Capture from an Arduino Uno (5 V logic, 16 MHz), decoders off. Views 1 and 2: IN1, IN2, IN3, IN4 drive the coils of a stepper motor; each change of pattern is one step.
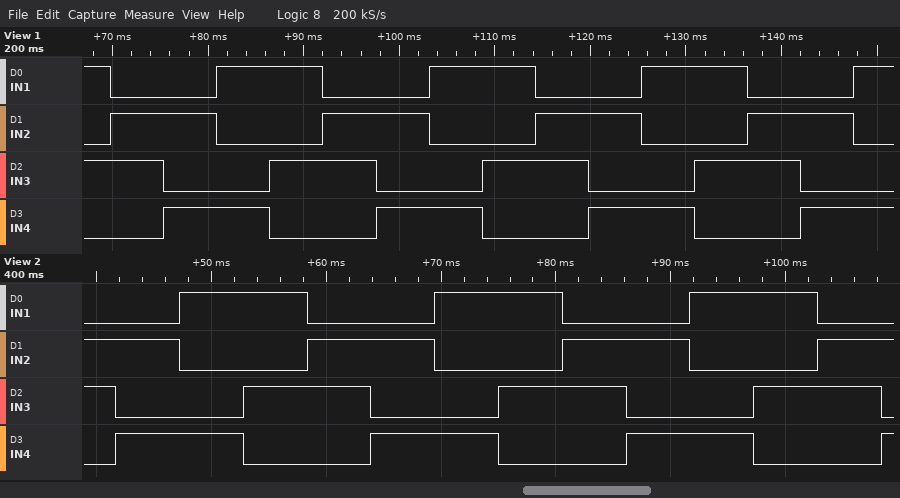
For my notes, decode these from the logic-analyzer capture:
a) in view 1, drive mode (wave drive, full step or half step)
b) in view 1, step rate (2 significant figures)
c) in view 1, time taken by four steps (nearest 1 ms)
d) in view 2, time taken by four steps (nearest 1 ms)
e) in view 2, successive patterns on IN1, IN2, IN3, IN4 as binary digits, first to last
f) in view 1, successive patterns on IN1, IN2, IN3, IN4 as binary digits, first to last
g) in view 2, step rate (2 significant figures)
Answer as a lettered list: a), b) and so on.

a) full step
b) 180 steps/s
c) 22 ms
d) 22 ms
e) 0110 0101 1001 1010 0110 0101 1001 1010 0110 0101 1001 1010 0110 0101
f) 1010 0110 0101 1001 1010 0110 0101 1001 1010 0110 0101 1001 1010 0110 0101 1001
g) 180 steps/s
